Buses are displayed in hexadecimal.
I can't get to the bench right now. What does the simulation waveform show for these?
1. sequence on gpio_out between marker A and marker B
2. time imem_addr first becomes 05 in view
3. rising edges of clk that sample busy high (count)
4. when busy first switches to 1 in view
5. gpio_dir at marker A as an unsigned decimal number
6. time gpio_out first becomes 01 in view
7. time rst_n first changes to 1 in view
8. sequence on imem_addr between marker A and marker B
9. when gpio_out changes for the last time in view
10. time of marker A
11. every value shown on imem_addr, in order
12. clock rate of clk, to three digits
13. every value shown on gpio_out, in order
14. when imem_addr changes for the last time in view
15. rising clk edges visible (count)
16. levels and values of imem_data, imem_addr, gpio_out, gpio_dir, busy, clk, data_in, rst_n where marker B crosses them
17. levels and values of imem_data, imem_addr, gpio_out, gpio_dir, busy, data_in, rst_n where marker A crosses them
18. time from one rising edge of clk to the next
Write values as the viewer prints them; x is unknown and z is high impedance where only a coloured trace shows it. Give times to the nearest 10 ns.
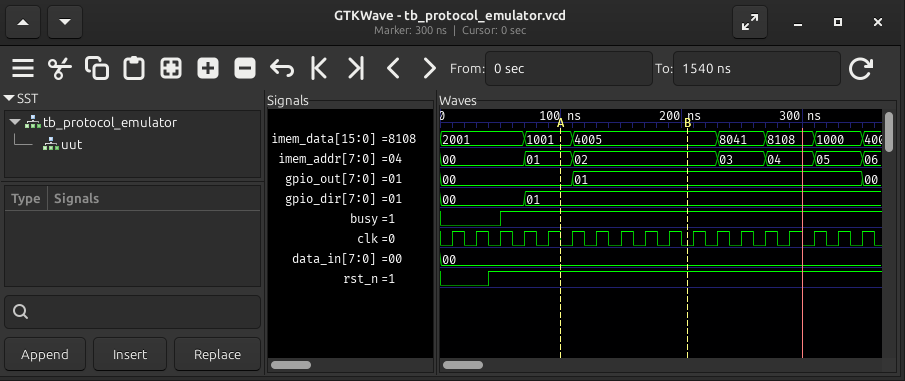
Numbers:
00, 01
310 ns
15
50 ns
1
110 ns
40 ns
01, 02
350 ns
100 ns
00, 01, 02, 03, 04, 05, 06
50.0 MHz
00, 01, 00
350 ns
18
imem_data=4005, imem_addr=02, gpio_out=01, gpio_dir=01, busy=1, clk=0, data_in=00, rst_n=1
imem_data=1001, imem_addr=01, gpio_out=00, gpio_dir=01, busy=1, data_in=00, rst_n=1
20 ns
